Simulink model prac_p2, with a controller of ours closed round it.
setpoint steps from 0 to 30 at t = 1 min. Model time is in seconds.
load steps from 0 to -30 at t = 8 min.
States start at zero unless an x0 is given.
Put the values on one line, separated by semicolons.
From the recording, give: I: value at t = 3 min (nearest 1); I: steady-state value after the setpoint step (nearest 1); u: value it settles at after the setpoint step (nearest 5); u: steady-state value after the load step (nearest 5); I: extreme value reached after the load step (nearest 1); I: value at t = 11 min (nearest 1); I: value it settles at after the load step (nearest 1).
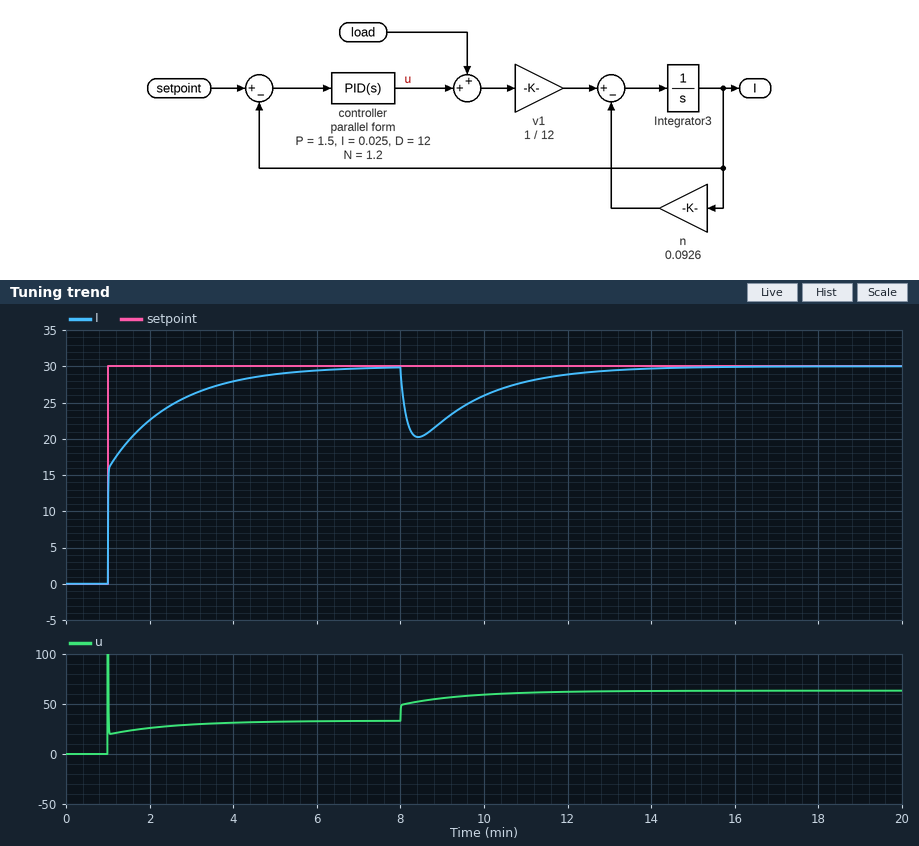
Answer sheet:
26; 30; 35; 65; 20; 28; 30
